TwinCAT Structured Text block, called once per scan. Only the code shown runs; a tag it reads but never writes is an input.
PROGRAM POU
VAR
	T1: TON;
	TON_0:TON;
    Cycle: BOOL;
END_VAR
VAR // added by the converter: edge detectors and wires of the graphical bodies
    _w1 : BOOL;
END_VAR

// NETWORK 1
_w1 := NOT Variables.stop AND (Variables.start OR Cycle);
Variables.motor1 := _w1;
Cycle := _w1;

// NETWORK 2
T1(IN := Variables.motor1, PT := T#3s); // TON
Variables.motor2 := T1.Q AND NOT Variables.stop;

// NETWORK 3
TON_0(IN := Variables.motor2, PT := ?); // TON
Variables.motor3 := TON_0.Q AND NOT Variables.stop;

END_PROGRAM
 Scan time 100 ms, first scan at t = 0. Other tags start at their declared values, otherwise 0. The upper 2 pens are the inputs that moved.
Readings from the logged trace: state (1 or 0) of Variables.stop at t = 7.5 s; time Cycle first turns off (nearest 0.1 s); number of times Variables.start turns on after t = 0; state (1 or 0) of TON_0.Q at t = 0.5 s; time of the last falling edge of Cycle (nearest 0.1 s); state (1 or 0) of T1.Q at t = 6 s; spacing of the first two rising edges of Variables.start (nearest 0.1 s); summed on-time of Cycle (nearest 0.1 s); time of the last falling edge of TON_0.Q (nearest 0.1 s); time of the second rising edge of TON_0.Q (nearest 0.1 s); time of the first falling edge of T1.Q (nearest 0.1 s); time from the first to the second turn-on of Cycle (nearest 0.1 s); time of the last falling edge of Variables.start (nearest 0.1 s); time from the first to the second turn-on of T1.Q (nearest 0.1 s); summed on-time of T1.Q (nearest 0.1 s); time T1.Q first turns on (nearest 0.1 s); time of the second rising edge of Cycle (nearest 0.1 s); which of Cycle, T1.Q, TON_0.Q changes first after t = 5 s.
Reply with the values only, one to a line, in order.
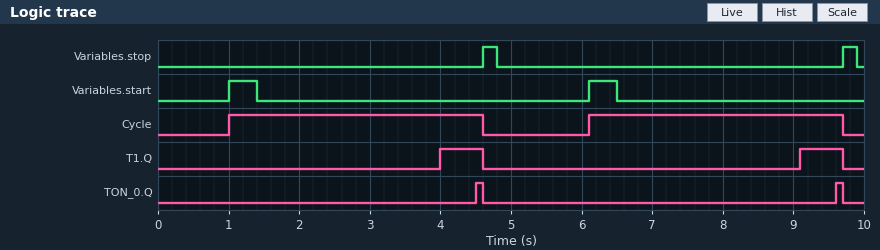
0
4.6 s
2
0
9.7 s
0
5.1 s
7.2 s
9.7 s
9.6 s
4.6 s
5.1 s
6.5 s
5.1 s
1.2 s
4.0 s
6.1 s
Cycle
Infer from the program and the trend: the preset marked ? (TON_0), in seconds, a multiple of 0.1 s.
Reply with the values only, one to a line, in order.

0.5 s
